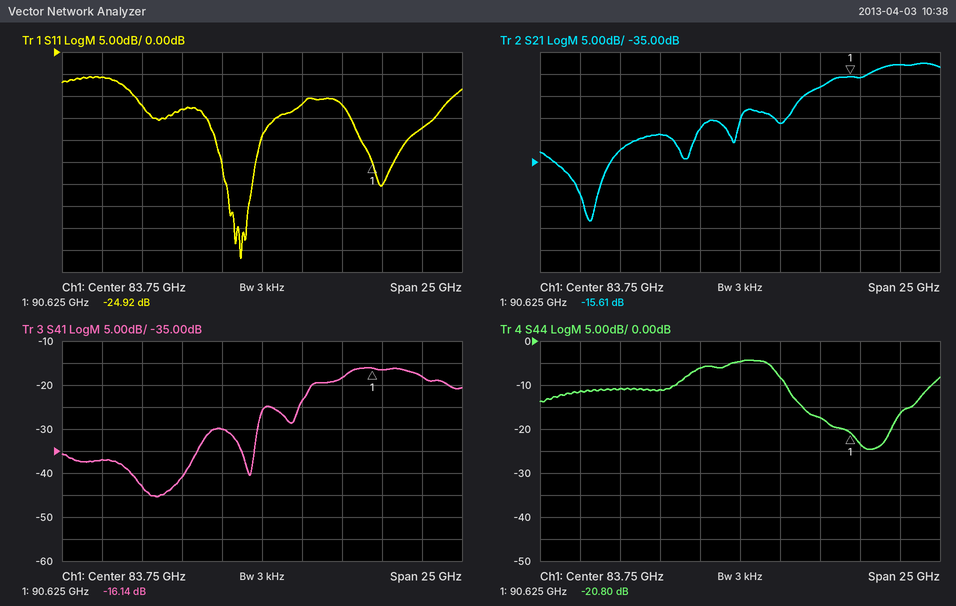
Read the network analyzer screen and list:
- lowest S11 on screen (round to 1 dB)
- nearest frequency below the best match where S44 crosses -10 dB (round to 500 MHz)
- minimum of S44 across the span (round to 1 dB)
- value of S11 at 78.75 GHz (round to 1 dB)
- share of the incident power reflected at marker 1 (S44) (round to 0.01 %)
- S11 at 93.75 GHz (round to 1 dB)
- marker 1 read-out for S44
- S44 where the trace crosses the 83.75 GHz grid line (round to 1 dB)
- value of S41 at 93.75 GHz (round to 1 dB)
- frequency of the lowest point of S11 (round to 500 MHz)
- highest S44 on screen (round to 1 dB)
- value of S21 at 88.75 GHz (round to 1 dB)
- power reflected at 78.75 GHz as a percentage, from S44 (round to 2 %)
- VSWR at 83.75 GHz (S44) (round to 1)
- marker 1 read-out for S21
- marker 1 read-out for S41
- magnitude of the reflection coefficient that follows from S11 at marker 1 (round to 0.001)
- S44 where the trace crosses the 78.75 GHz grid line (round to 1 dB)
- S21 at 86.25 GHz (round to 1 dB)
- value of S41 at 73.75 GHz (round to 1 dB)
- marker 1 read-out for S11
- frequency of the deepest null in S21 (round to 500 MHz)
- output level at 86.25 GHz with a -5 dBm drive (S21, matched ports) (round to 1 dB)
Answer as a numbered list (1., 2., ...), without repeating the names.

1. -47 dB
2. 86.5 GHz
3. -25 dB
4. -13 dB
5. 0.83 %
6. -17 dB
7. -20.80 dB
8. -5 dB
9. -18 dB
10. 82.5 GHz
11. -4 dB
12. -18 dB
13. 8 %
14. 4
15. -15.61 dB
16. -16.14 dB
17. 0.057
18. -11 dB
19. -26 dB
20. -37 dB
21. -24.92 dB
22. 74.5 GHz
23. -31 dBm
